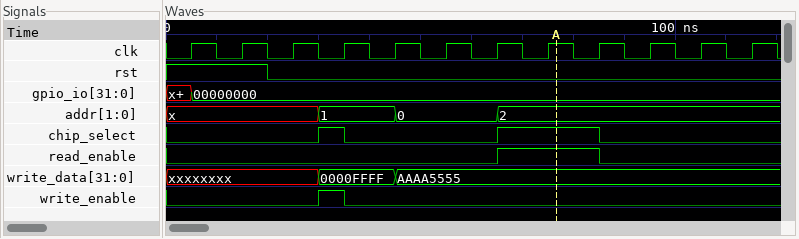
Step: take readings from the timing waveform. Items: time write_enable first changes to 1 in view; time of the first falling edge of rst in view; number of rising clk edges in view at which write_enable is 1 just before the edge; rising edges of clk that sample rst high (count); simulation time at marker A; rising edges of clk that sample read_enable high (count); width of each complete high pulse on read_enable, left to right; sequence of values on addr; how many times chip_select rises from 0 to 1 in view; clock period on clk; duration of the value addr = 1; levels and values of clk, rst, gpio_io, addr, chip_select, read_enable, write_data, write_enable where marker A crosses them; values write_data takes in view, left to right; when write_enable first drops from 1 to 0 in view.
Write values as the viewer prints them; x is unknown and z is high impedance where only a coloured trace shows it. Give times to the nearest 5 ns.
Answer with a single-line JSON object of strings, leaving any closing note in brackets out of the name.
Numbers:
{"time write_enable first changes to 1 in view": "30 ns", "time of the first falling edge of rst in view": "20 ns", "number of rising clk edges in view at which write_enable is 1 just before the edge": "1", "rising edges of clk that sample rst high": "2", "simulation time at marker A": "75 ns", "rising edges of clk that sample read_enable high": "2", "width of each complete high pulse on read_enable, left to right": "20 ns", "sequence of values on addr": "x, 1, 0, 2", "how many times chip_select rises from 0 to 1 in view": "2", "clock period on clk": "10 ns", "duration of the value addr = 1": "15 ns", "levels and values of clk, rst, gpio_io, addr, chip_select, read_enable, write_data, write_enable where marker A crosses them": "clk=1, rst=0, gpio_io=00000000, addr=2, chip_select=1, read_enable=1, write_data=AAAA5555, write_enable=0", "values write_data takes in view, left to right": "xxxxxxxx, 0000FFFF, AAAA5555", "when write_enable first drops from 1 to 0 in view": "35 ns"}
